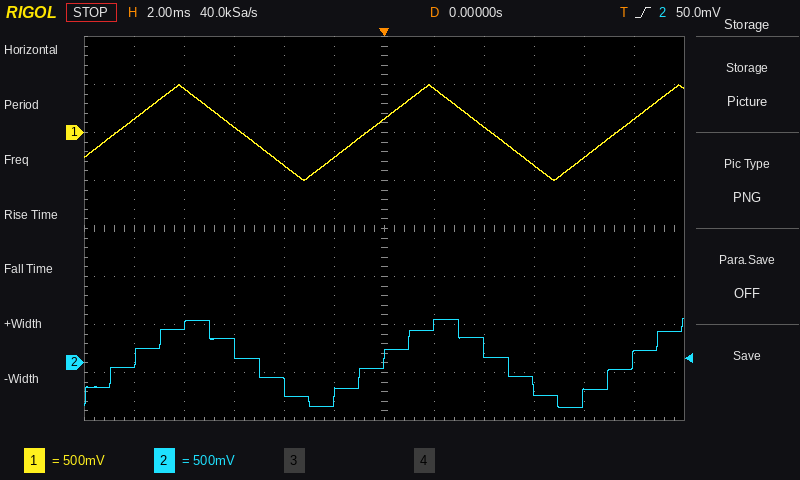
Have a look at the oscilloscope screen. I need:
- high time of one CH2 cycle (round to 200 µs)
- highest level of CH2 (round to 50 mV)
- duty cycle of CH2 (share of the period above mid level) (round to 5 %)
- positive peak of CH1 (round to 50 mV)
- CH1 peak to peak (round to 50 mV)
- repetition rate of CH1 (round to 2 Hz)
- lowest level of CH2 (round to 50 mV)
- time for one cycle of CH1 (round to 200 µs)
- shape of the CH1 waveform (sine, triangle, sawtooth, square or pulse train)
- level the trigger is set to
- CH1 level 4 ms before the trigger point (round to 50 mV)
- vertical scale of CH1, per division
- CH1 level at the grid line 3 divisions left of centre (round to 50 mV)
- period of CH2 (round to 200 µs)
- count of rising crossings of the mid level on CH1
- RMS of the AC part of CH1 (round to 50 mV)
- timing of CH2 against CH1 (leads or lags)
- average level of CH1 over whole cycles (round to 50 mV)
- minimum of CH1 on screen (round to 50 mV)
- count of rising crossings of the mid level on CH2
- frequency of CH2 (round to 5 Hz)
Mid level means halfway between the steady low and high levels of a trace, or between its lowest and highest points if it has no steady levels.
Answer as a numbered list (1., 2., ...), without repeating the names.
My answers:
1. 5.0 ms
2. 450 mV
3. 50 %
4. 500 mV
5. 1.00 V
6. 100 Hz
7. -450 mV
8. 10.0 ms
9. triangle
10. 50.0 mV
11. -350 mV
12. 500 mV
13. 50 mV
14. 10.0 ms
15. 3
16. 300 mV
17. lags
18. 0 mV
19. -500 mV
20. 3
21. 100 Hz
